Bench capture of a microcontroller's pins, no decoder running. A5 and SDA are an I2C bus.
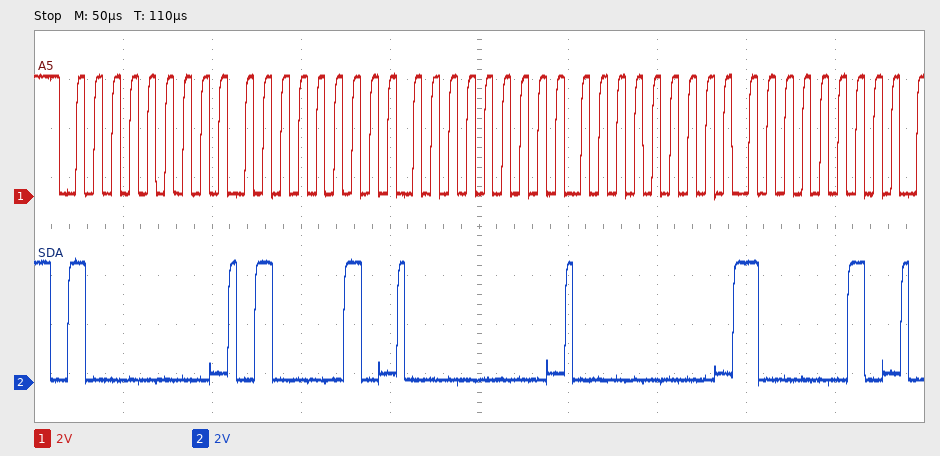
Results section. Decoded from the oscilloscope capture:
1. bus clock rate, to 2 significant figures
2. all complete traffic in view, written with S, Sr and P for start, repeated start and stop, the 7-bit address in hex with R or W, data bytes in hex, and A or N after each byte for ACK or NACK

100 kHz
S 40W A 42 A 00 A 00 A 82 A
